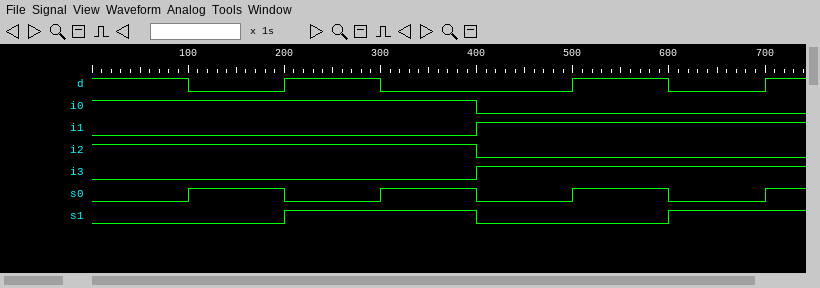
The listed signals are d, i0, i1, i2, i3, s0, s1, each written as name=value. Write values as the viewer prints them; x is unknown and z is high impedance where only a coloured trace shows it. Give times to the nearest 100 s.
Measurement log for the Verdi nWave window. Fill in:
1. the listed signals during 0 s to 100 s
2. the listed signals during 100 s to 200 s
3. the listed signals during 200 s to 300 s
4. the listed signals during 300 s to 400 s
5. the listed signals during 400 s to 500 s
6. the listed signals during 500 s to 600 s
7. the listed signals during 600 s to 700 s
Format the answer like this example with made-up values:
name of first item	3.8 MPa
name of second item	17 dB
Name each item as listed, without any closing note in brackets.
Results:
the listed signals during 0 s to 100 s	d=1, i0=1, i1=0, i2=1, i3=0, s0=0, s1=0
the listed signals during 100 s to 200 s	d=0, i0=1, i1=0, i2=1, i3=0, s0=1, s1=0
the listed signals during 200 s to 300 s	d=1, i0=1, i1=0, i2=1, i3=0, s0=0, s1=1
the listed signals during 300 s to 400 s	d=0, i0=1, i1=0, i2=1, i3=0, s0=1, s1=1
the listed signals during 400 s to 500 s	d=0, i0=0, i1=1, i2=0, i3=1, s0=0, s1=0
the listed signals during 500 s to 600 s	d=1, i0=0, i1=1, i2=0, i3=1, s0=1, s1=0
the listed signals during 600 s to 700 s	d=0, i0=0, i1=1, i2=0, i3=1, s0=0, s1=1
